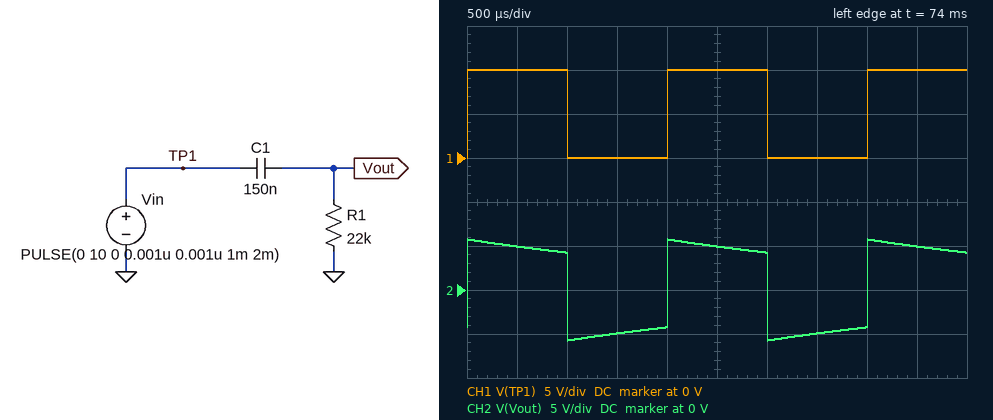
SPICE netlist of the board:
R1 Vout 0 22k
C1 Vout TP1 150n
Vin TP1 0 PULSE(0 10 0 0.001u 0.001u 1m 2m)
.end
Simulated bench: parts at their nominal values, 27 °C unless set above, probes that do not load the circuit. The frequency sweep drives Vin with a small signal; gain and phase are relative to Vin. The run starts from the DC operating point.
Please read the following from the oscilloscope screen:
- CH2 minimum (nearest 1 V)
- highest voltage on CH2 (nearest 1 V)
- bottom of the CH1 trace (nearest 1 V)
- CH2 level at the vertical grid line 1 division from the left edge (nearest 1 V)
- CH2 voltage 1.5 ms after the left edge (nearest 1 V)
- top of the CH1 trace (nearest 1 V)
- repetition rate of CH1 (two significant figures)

-6 V
6 V
0 V
5 V
-5 V
10 V
500 Hz
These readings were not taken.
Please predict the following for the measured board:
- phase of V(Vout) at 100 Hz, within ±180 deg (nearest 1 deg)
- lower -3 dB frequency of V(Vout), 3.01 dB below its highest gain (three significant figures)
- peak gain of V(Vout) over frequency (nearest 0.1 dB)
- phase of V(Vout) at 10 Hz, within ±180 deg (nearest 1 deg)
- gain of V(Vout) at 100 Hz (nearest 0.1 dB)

26 deg
48.2 Hz
0 dB
78 deg
-0.9 dB
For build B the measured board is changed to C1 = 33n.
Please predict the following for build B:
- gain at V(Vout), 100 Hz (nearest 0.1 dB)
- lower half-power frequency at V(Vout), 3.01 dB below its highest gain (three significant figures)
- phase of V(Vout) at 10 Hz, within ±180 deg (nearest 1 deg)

-7.6 dB
219 Hz
87 deg
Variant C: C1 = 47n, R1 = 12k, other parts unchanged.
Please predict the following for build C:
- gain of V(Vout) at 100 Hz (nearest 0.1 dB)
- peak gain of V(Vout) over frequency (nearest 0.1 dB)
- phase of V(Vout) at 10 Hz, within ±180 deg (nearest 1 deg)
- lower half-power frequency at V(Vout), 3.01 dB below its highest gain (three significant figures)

-9.5 dB
0 dB
88 deg
282 Hz
